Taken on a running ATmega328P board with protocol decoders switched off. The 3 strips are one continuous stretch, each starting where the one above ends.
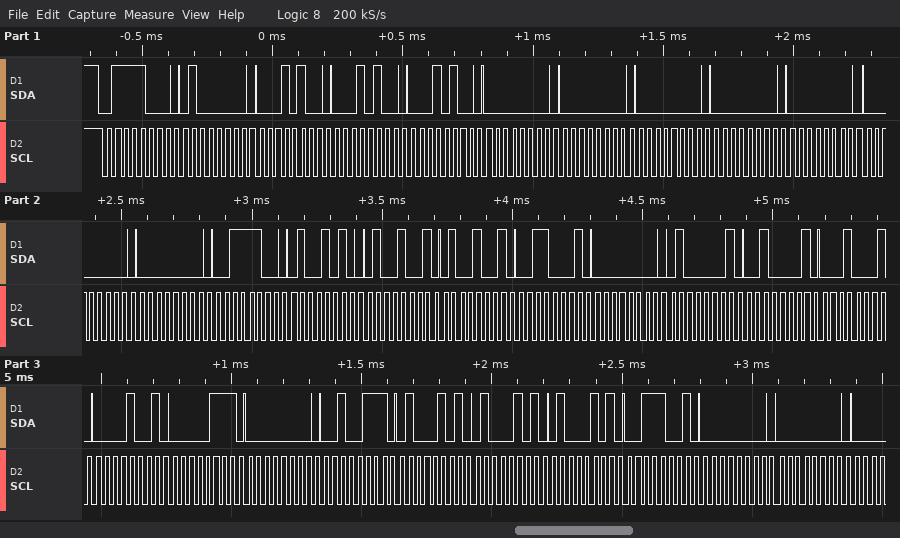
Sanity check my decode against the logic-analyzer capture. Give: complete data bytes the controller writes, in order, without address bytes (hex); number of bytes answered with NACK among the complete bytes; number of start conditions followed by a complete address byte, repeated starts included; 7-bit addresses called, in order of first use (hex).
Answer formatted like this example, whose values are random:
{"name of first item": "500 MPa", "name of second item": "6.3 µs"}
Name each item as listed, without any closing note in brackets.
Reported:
{"complete data bytes the controller writes, in order, without address bytes": "40 14 14 14 00 00 00 00 00 00 00 3C 4A 49 49 31 00 41 21 11 09 07 00 27 45 45 45 39 00 00", "number of bytes answered with NACK among the complete bytes": "0", "number of start conditions followed by a complete address byte, repeated starts included": "1", "7-bit addresses called, in order of first use": "0x3C"}
